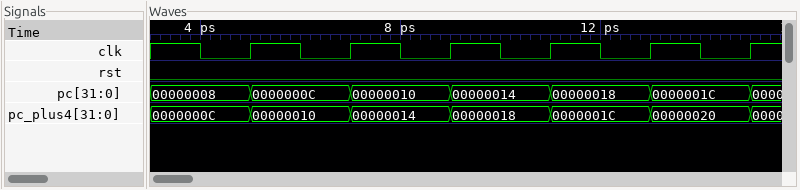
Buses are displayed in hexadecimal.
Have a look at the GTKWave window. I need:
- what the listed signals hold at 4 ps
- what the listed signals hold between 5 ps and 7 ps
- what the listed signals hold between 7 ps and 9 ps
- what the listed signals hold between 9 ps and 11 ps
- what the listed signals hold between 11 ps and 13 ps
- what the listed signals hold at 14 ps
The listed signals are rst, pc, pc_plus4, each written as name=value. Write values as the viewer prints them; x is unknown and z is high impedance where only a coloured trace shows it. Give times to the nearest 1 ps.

rst=0, pc=00000008, pc_plus4=0000000C
rst=0, pc=0000000C, pc_plus4=00000010
rst=0, pc=00000010, pc_plus4=00000014
rst=0, pc=00000014, pc_plus4=00000018
rst=0, pc=00000018, pc_plus4=0000001C
rst=0, pc=0000001C, pc_plus4=00000020
